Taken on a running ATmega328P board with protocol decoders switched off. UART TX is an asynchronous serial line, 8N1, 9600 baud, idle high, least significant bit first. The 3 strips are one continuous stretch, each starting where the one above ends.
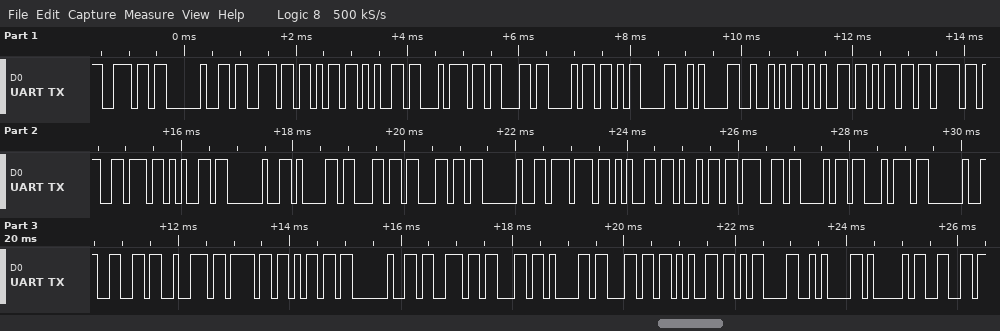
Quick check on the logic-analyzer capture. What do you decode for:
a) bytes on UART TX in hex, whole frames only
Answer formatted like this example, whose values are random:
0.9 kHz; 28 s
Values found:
0x6E 0x20 0x73 0x6B 0x65 0x74 0x63 0x68 0x0D 0x0A 0x52 0x65 0x6D 0x6F 0x76 0x65 0x20 0x61 0x6C 0x6C 0x20 0x77 0x65 0x69 0x67 0x68 0x74 0x20 0x66 0x72 0x6F 0x6D 0x20 0x73 0x63 0x61 0x6C 0x65 0x0D 0x0A 0x41 0x66
